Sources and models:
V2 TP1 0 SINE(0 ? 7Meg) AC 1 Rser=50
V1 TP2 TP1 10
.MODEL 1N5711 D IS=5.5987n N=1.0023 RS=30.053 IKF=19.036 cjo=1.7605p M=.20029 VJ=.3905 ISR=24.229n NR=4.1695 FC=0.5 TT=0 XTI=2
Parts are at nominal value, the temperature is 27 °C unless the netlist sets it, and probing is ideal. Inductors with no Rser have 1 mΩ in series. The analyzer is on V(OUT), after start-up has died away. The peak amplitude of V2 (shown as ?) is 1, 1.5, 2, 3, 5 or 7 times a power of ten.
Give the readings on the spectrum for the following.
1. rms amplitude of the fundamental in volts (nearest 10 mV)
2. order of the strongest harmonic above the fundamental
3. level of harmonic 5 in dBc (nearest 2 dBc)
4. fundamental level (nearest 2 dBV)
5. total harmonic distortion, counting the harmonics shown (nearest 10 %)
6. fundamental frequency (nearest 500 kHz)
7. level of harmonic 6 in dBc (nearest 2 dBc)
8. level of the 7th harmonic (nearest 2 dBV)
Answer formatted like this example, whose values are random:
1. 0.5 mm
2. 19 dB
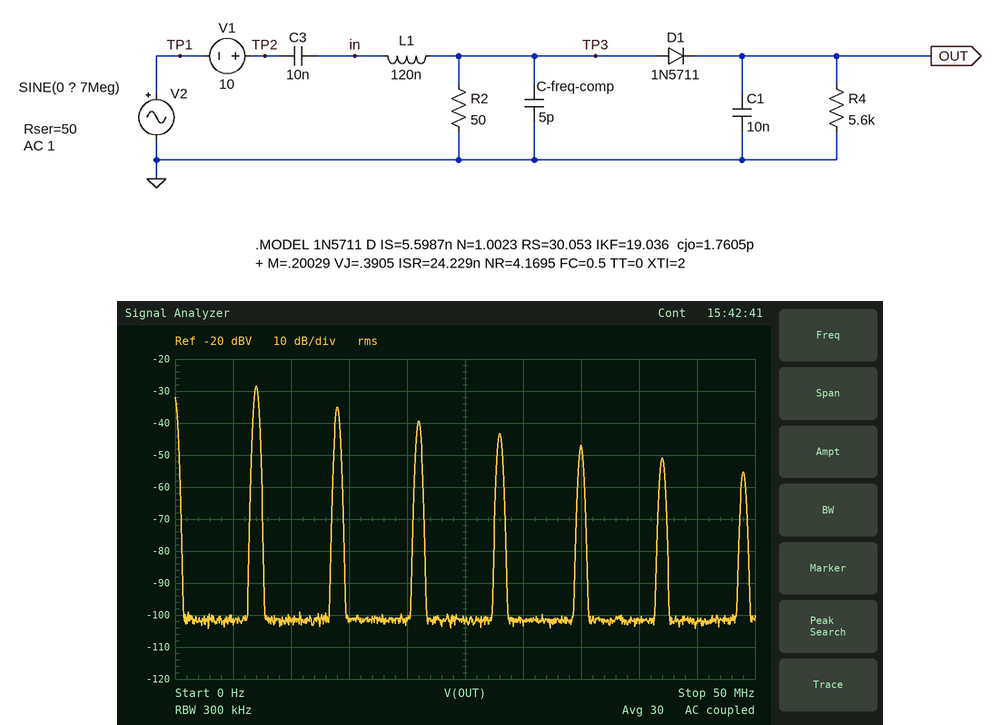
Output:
1. 40 mV
2. 2
3. -18 dBc
4. -28 dBV
5. 60 %
6. 7.0 MHz
7. -22 dBc
8. -56 dBV
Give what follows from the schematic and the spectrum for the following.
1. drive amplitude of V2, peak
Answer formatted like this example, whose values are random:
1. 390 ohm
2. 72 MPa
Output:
1. 150 V
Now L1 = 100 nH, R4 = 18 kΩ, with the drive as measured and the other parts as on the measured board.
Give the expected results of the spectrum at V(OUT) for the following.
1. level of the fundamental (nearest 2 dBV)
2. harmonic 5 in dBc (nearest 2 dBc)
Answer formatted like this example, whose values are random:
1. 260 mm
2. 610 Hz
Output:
1. -38 dBV
2. -16 dBc
